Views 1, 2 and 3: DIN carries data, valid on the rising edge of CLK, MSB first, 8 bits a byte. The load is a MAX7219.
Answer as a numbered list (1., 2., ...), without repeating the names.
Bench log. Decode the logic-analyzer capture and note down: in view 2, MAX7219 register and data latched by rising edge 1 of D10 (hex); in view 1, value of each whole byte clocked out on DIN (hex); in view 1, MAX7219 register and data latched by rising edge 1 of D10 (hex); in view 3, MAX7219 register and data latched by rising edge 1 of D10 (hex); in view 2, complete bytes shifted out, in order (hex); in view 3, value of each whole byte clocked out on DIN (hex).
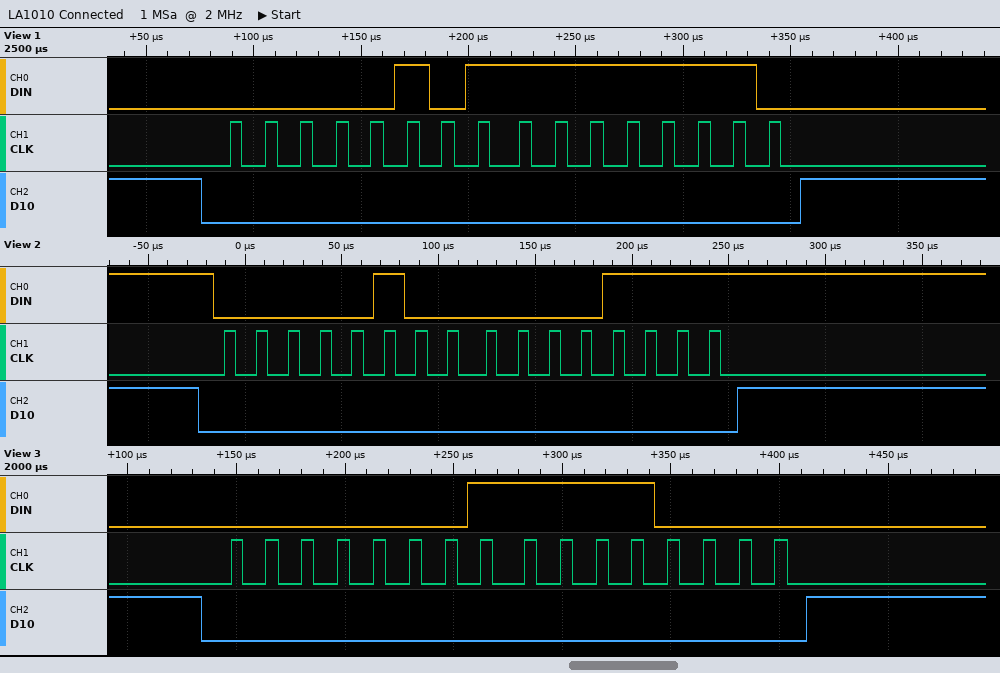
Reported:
1. register 0x4, data 0x0F
2. 05 FE
3. register 0x5, data 0xFE
4. register 0x1, data 0xF0
5. 04 0F
6. 0x01 0xF0
